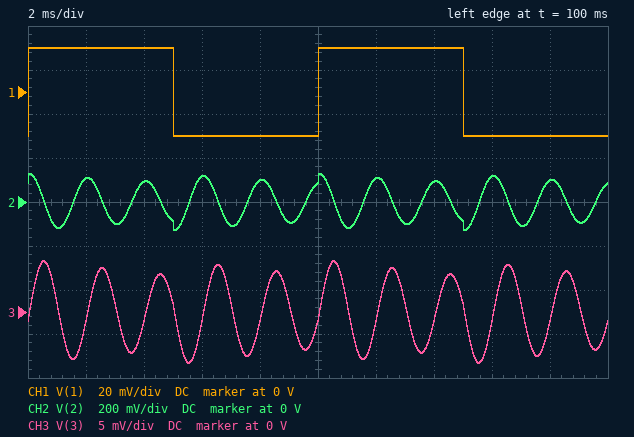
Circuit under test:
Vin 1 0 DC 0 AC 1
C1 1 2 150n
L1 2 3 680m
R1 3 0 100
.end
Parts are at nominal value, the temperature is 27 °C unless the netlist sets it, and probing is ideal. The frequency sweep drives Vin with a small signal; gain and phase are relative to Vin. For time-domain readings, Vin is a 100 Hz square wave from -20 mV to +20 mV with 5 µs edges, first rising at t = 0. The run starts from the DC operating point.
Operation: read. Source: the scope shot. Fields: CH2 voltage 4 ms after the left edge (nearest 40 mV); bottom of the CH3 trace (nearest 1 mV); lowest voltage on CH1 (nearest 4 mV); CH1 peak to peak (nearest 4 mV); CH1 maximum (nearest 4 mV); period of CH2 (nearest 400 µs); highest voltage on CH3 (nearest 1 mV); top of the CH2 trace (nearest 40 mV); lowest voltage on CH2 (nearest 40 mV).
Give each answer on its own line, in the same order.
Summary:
80 mV
-6 mV
-20 mV
40 mV
20 mV
2.0 ms
6 mV
120 mV
-120 mV
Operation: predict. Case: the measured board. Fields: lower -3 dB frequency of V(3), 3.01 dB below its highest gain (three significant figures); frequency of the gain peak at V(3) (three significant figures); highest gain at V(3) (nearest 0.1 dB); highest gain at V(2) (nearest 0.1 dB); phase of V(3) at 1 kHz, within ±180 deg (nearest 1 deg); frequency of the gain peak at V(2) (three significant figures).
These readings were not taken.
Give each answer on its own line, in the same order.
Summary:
487 Hz
498 Hz
0 dB
26.6 dB
-88 deg
499 Hz
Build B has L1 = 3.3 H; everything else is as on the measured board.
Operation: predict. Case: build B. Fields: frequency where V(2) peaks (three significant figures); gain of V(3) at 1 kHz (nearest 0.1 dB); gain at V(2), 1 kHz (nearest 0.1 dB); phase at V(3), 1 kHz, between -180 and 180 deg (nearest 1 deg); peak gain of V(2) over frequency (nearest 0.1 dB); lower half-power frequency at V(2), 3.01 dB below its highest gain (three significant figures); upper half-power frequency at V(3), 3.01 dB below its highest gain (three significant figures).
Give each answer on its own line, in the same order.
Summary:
226 Hz
-45.9 dB
0.5 dB
-90 deg
33.4 dB
224 Hz
229 Hz
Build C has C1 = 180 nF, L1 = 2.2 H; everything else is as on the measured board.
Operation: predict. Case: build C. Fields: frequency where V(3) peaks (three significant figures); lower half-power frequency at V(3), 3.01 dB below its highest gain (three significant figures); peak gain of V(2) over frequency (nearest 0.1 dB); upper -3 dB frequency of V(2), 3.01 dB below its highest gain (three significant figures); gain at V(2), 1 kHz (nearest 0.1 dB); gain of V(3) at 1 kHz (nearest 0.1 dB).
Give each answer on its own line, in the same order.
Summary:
253 Hz
249 Hz
30.9 dB
257 Hz
0.6 dB
-42.2 dB
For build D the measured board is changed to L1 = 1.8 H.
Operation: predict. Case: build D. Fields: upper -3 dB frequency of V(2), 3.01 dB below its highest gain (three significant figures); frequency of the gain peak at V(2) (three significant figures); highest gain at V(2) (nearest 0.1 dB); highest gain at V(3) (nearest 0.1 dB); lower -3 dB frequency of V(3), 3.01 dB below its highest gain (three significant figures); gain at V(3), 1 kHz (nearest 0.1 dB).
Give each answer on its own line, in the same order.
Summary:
311 Hz
306 Hz
30.8 dB
0 dB
302 Hz
-40.2 dB
